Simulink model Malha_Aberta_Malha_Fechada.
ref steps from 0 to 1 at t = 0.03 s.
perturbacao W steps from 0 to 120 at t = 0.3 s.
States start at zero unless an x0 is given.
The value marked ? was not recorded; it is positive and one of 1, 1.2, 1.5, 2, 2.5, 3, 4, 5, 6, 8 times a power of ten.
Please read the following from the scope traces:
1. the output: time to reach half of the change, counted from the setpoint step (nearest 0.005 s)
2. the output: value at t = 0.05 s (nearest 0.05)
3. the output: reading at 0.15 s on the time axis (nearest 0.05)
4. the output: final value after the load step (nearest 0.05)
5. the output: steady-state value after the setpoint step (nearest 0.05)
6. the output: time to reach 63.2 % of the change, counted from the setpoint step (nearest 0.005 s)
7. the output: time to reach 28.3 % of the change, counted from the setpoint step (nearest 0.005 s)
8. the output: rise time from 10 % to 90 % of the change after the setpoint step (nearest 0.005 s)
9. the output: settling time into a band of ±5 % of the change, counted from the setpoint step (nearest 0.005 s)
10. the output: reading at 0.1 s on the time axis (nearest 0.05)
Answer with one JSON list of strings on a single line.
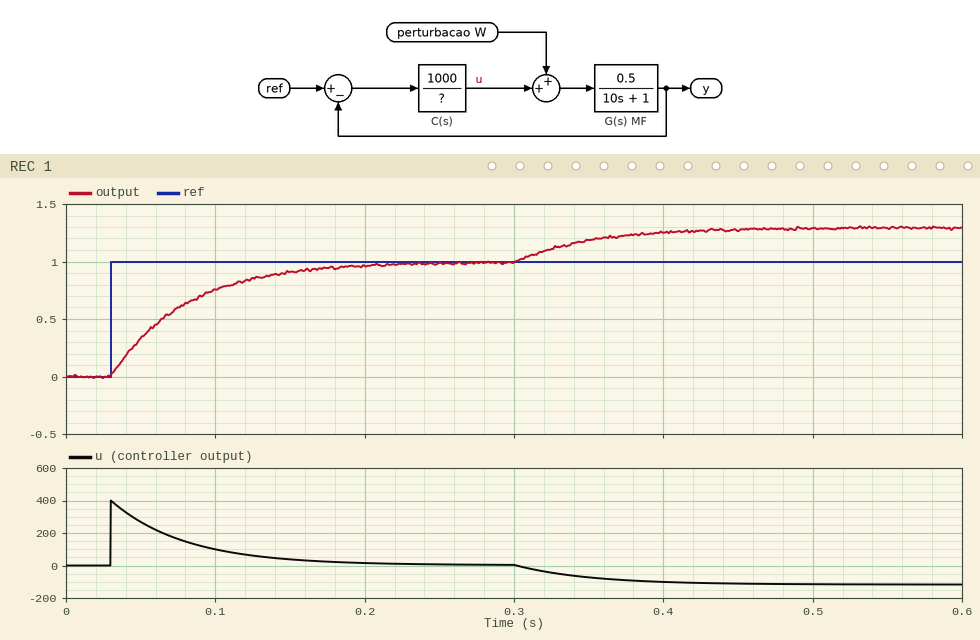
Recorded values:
["0.035 s", "0.35", "0.90", "1.30", "1.00", "0.050 s", "0.015 s", "0.110 s", "0.150 s", "0.75"]
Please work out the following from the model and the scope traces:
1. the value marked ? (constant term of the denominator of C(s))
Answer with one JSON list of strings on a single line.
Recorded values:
["2.5"]
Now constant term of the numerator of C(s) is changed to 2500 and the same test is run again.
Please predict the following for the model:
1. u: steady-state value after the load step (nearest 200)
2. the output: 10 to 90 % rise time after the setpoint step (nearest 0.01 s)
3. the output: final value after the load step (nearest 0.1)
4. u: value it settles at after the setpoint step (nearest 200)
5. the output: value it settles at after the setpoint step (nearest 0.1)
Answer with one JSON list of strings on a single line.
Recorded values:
["-200", "0.04 s", "1.1", "0", "1.0"]
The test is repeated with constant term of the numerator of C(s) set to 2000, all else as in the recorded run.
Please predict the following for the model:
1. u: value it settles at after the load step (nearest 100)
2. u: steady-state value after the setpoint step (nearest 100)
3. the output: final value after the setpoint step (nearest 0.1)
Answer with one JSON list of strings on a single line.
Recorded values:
["-100", "0", "1.0"]
